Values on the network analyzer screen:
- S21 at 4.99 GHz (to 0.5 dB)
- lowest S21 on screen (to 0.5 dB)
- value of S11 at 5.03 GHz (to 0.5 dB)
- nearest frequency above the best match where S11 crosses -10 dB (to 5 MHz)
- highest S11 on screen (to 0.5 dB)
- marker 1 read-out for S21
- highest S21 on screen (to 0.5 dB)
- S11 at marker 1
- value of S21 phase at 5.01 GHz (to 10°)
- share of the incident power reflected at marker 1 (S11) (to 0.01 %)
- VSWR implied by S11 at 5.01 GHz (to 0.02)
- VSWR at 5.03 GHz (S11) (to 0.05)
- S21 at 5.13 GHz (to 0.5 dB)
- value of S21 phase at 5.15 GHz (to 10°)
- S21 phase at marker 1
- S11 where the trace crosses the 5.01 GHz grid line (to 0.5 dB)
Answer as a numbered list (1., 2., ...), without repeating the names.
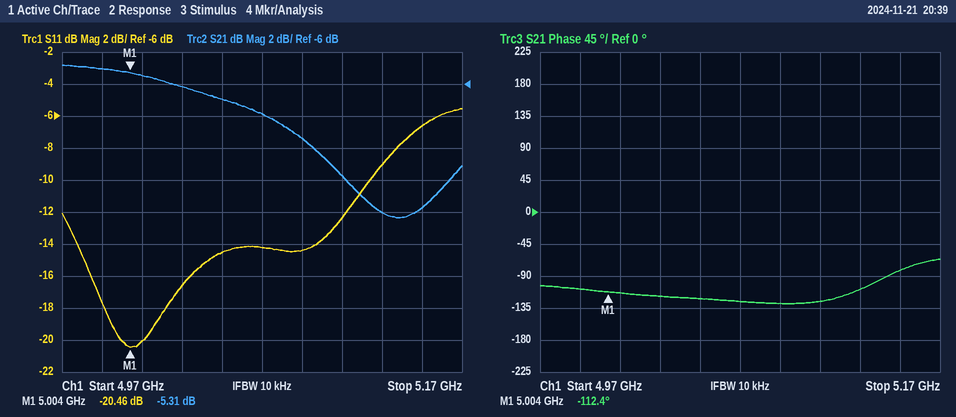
1. -5.0 dB
2. -14.5 dB
3. -16.5 dB
4. 5.125 GHz
5. -5.5 dB
6. -5.31 dB
7. -5.0 dB
8. -20.46 dB
9. -110°
10. 0.90 %
11. 1.22
12. 1.35
13. -14.0 dB
14. -80°
15. -112.4°
16. -20.0 dB
